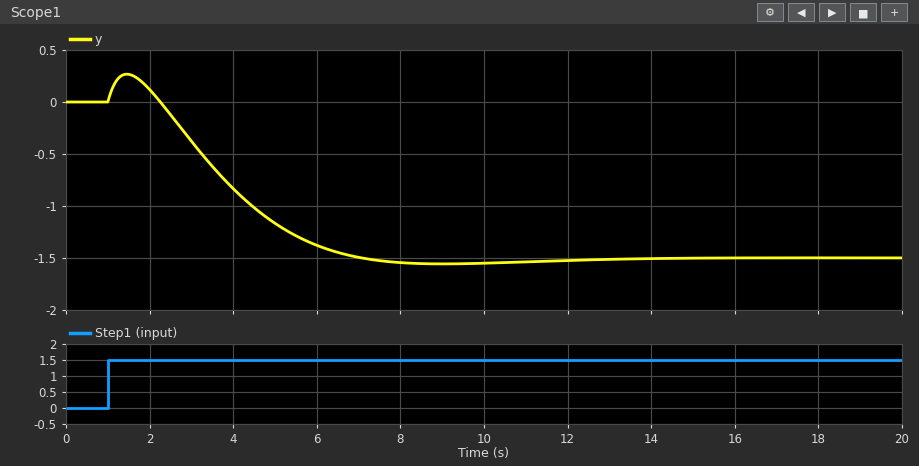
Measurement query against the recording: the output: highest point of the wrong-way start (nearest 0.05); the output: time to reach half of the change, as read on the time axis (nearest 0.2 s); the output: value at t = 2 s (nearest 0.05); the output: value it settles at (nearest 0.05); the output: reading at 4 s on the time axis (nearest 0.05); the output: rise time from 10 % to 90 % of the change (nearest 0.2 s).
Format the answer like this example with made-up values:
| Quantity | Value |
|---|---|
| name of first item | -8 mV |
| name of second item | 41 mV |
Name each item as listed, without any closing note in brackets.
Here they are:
| Quantity | Value |
|---|---|
| the output: highest point of the wrong-way start | 0.25 |
| the output: time to reach half of the change, as read on the time axis | 3.8 s |
| the output: value at t = 2 s | 0.10 |
| the output: value it settles at | -1.50 |
| the output: reading at 4 s on the time axis | -0.85 |
| the output: rise time from 10 % to 90 % of the change | 3.2 s |
